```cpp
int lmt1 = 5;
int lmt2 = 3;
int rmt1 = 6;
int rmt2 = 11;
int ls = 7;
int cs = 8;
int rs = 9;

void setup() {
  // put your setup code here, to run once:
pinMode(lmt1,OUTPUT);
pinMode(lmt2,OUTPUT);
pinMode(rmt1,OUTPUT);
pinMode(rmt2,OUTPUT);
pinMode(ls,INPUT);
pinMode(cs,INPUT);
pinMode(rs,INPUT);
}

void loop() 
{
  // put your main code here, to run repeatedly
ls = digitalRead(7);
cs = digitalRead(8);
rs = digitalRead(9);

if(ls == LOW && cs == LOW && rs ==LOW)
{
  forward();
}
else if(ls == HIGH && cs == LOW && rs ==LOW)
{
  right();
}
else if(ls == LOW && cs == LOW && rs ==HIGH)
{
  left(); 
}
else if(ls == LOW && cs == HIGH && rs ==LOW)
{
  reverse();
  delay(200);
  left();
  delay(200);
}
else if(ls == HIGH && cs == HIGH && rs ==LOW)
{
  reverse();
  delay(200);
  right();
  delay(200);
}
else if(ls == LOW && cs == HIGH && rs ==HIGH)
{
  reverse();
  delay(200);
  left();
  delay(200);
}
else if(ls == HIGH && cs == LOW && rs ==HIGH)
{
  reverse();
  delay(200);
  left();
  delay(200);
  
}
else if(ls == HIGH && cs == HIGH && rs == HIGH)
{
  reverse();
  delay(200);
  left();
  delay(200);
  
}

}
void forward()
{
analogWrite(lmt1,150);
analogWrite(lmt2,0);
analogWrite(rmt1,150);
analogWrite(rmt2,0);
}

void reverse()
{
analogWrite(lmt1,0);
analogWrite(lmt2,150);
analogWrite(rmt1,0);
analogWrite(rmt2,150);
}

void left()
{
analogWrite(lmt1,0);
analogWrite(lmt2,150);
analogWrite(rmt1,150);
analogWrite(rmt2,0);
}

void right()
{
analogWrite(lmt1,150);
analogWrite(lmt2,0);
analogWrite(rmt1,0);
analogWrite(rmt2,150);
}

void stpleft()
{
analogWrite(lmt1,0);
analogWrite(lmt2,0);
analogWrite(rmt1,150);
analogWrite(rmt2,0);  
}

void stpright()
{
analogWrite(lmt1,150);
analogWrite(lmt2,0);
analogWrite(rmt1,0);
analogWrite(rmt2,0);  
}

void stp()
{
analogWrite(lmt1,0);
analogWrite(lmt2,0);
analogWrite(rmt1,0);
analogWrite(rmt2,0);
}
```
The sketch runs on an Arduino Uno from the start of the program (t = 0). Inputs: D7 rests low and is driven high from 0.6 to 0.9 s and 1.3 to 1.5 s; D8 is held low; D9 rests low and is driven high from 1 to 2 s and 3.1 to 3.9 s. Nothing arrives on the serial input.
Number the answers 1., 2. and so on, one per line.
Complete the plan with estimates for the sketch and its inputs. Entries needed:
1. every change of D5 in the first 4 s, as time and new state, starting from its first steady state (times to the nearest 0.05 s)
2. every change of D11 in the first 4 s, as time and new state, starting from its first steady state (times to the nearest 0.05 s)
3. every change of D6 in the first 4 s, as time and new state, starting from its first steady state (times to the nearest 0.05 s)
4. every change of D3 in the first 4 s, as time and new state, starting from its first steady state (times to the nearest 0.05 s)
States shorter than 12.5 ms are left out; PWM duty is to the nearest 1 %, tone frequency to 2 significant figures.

1. 0 s PWM 59 %; 1 s low; 2 s PWM 59 %; 3.1 s low; 3.9 s PWM 59 %
2. 0 s low; 0.6 s PWM 59 %; 0.9 s low; 1.3 s PWM 59 %; 1.5 s low
3. 0 s PWM 59 %; 0.6 s low; 0.9 s PWM 59 %; 1.3 s low; 1.5 s PWM 59 %
4. 0 s low; 1 s PWM 59 %; 2 s low; 3.1 s PWM 59 %; 3.9 s low
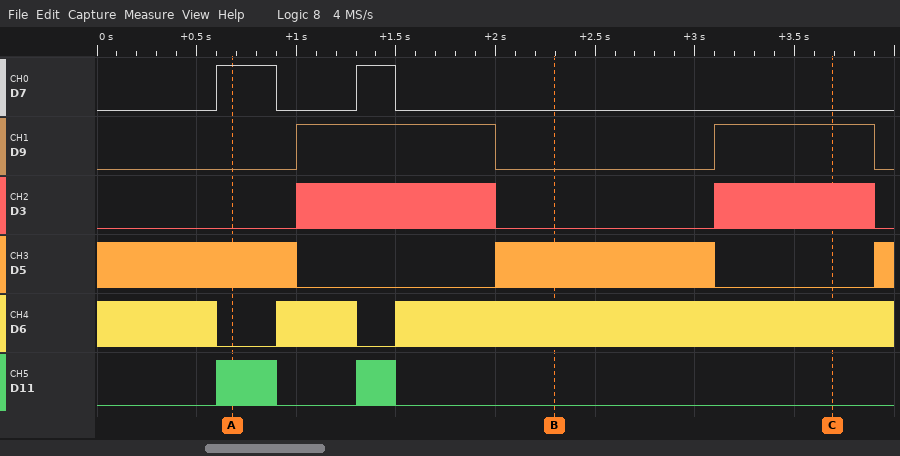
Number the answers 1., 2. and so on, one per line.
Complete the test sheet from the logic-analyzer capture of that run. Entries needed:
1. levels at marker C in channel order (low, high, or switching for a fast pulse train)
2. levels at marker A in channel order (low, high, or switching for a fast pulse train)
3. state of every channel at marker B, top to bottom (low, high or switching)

1. D7 low, D9 high, D3 switching, D5 low, D6 switching, D11 low
2. D7 high, D9 low, D3 low, D5 switching, D6 low, D11 switching
3. D7 low, D9 low, D3 low, D5 switching, D6 switching, D11 low
